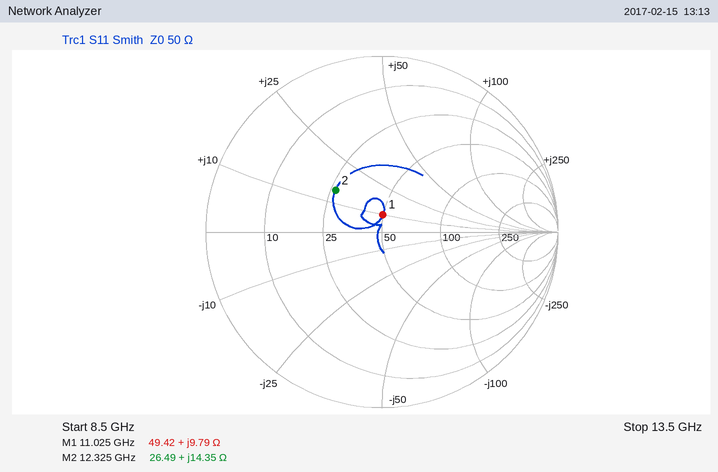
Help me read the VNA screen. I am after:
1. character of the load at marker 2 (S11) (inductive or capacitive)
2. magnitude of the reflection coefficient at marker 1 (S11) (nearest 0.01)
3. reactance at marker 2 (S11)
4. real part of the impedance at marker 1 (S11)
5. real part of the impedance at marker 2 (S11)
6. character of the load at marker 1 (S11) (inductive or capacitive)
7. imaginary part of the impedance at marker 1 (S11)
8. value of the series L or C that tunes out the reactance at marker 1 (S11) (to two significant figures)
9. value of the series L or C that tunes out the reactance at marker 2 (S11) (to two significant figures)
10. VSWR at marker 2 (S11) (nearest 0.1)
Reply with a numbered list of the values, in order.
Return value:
1. inductive
2. 0.10
3. +14.35 Ω
4. 49.42 Ω
5. 26.49 Ω
6. inductive
7. +9.79 Ω
8. 1.5 pF
9. 900 fF
10. 2.1
